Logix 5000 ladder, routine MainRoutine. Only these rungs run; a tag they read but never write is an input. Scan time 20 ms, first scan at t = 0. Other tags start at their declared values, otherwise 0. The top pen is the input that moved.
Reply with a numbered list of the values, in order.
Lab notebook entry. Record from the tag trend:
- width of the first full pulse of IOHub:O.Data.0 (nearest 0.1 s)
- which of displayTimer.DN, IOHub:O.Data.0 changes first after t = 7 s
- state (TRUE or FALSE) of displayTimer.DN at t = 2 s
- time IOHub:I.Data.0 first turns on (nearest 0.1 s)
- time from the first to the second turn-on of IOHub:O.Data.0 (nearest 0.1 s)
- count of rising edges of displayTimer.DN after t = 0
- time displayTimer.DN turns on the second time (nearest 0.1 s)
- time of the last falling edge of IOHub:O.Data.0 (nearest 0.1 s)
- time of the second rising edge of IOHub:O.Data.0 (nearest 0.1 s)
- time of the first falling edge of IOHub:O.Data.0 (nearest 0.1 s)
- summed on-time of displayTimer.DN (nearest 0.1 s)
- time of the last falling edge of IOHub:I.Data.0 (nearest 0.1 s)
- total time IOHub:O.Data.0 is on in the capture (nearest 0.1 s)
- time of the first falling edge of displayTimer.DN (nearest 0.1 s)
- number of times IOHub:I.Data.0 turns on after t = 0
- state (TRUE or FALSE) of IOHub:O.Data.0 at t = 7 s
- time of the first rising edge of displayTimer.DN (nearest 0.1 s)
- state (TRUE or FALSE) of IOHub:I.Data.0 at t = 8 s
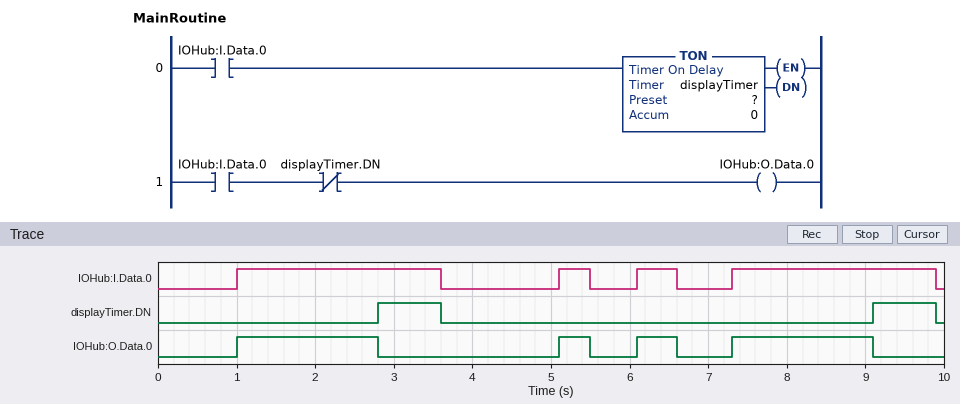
1. 1.8 s
2. IOHub:O.Data.0
3. FALSE
4. 1.0 s
5. 4.1 s
6. 2
7. 9.1 s
8. 9.1 s
9. 5.1 s
10. 2.8 s
11. 1.6 s
12. 9.9 s
13. 4.5 s
14. 3.6 s
15. 4
16. FALSE
17. 2.8 s
18. TRUE
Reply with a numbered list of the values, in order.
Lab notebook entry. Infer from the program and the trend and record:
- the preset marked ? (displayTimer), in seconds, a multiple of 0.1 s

1. 1.8 s
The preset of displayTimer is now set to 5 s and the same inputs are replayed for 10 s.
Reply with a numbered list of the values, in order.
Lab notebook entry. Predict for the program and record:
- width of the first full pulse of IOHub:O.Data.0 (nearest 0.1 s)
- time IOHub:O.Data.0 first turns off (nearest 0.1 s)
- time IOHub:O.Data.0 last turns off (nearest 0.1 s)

1. 2.6 s
2. 3.6 s
3. 9.9 s
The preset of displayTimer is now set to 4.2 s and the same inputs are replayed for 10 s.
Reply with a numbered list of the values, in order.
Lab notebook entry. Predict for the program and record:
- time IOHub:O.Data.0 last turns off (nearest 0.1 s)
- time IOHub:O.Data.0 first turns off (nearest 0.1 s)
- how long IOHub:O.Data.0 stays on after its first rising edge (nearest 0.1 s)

1. 9.9 s
2. 3.6 s
3. 2.6 s
